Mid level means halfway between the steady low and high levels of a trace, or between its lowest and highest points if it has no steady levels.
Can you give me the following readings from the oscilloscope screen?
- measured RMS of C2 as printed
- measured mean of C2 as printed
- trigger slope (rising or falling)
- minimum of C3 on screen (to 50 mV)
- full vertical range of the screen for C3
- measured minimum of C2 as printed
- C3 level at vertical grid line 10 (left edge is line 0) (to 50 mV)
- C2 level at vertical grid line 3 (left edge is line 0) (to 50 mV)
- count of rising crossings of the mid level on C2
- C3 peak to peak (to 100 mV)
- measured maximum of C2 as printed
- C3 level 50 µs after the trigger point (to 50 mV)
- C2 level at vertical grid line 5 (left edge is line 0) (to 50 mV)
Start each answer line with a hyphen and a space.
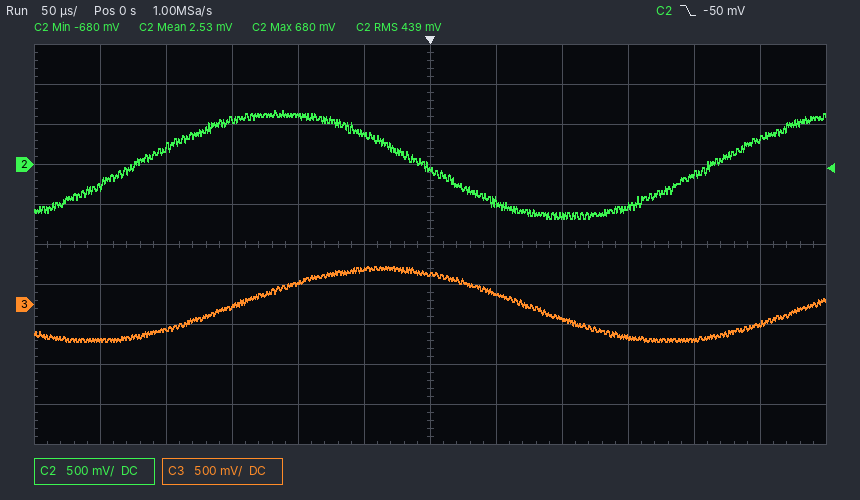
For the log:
- 439 mV
- 2.53 mV
- falling
- -450 mV
- 5 V
- -680 mV
- -450 mV
- 550 mV
- 2
- 900 mV
- 680 mV
- 150 mV
- 400 mV
